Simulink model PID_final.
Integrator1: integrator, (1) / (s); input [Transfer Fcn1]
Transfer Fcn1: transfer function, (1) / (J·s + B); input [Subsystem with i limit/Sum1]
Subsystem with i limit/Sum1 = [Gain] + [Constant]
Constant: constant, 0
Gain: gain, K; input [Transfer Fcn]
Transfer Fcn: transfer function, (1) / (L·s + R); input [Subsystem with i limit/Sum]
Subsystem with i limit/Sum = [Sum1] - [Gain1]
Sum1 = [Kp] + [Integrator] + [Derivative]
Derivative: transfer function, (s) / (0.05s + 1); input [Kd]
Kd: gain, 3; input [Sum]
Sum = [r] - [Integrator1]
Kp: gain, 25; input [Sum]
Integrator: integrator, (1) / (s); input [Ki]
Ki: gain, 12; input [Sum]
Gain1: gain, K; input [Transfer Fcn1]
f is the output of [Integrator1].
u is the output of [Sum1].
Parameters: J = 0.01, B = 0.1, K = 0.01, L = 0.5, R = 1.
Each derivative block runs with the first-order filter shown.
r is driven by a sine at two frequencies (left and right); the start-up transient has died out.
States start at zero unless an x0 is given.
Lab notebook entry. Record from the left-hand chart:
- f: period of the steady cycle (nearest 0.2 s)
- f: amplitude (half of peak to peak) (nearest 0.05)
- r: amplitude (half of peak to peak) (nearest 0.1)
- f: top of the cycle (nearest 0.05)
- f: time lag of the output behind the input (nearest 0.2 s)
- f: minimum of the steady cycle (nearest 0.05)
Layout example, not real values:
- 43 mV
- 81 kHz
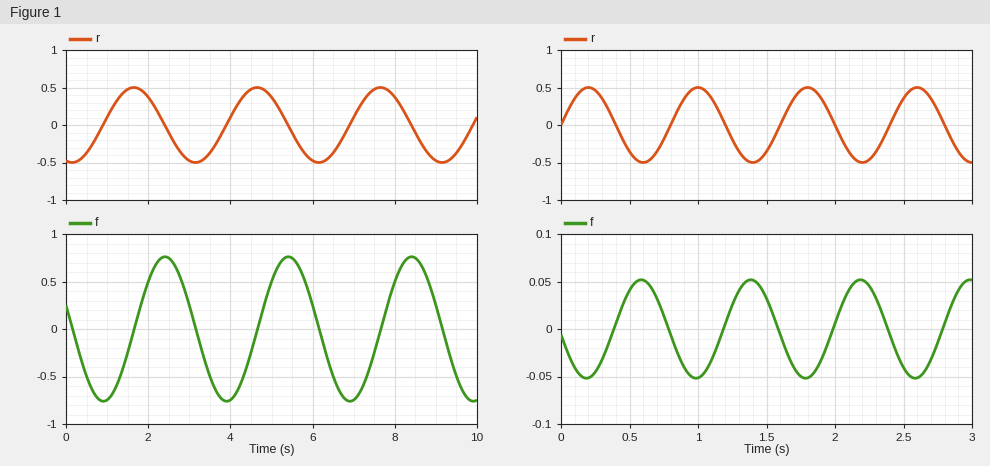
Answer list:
- 3.0 s
- 0.75
- 0.5
- 0.75
- 0.8 s
- -0.75
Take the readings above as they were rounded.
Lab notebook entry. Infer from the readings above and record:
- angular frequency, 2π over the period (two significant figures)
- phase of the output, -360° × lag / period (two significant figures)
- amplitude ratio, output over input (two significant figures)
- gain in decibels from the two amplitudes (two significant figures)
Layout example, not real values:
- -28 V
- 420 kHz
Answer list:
- 2.1 rad/s
- -96°
- 1.5
- 3.5 dB
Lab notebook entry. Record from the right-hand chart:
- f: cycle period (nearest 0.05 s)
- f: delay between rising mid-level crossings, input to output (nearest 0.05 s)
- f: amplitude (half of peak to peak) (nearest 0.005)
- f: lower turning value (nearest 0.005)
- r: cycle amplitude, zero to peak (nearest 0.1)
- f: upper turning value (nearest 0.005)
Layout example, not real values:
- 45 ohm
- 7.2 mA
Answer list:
- 0.80 s
- 0.40 s
- 0.050
- -0.050
- 0.5
- 0.050
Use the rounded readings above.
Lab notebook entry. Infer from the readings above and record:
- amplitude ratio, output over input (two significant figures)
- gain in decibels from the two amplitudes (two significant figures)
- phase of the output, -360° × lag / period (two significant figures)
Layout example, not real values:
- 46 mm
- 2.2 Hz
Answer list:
- 0.10
- -20 dB
- -180°
